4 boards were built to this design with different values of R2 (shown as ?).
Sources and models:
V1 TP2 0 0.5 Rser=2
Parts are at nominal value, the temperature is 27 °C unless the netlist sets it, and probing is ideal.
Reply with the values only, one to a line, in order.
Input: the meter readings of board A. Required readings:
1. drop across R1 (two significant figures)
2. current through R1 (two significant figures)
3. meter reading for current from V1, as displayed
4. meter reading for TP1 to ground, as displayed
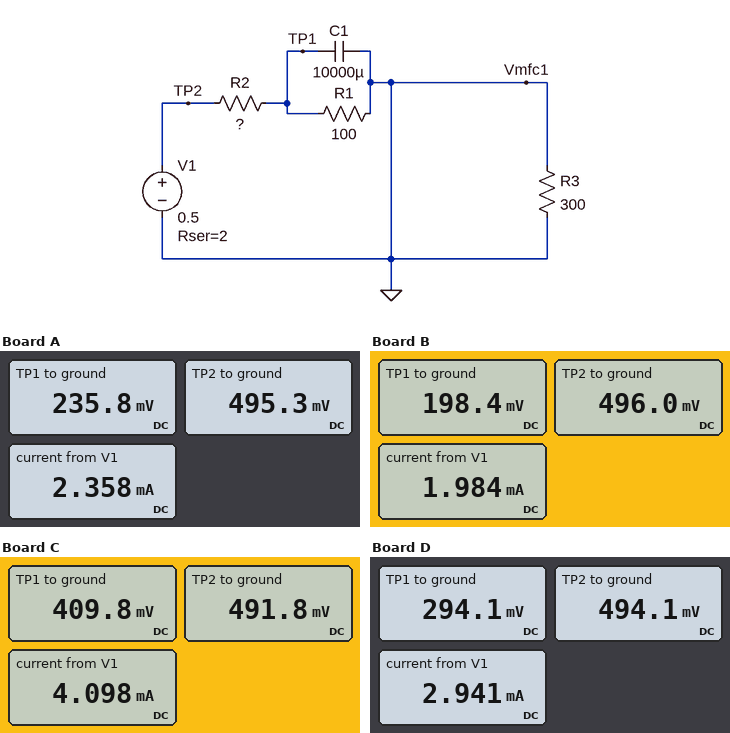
240 mV
2.4 mA
2.358 mA
235.8 mV
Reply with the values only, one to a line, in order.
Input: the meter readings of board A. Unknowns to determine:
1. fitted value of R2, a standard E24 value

110 Ω
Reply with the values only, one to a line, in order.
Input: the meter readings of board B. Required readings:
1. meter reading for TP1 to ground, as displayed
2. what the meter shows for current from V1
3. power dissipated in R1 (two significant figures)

198.4 mV
1.984 mA
390 µW
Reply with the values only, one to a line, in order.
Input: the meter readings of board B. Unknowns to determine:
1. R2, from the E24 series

150 Ω
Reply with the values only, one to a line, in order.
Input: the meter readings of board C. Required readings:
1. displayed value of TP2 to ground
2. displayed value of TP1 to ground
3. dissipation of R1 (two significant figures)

491.8 mV
409.8 mV
1.7 mW
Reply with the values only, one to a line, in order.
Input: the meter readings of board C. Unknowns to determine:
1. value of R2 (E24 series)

20 Ω
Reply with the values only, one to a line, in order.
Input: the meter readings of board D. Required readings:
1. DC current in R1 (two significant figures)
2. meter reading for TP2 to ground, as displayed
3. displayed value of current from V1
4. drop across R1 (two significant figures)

2.9 mA
494.1 mV
2.941 mA
290 mV
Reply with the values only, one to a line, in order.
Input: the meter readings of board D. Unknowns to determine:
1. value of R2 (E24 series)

68 Ω
